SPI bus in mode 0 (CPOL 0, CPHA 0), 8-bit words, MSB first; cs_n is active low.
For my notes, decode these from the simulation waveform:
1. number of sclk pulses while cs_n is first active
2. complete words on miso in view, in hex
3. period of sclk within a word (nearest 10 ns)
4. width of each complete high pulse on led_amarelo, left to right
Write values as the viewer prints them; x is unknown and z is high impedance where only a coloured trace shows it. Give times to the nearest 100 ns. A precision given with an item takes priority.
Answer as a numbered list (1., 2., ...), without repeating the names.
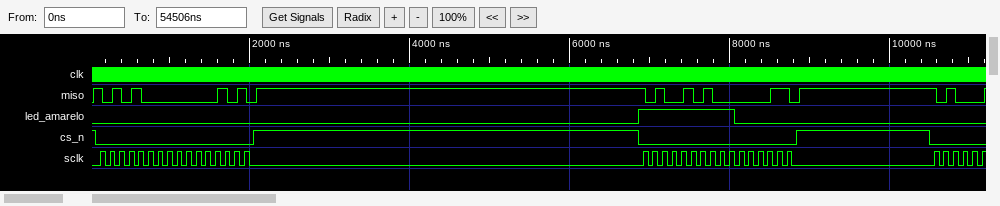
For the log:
1. 16
2. A8, 05, A5, 03
3. 120 ns
4. 1200 ns
